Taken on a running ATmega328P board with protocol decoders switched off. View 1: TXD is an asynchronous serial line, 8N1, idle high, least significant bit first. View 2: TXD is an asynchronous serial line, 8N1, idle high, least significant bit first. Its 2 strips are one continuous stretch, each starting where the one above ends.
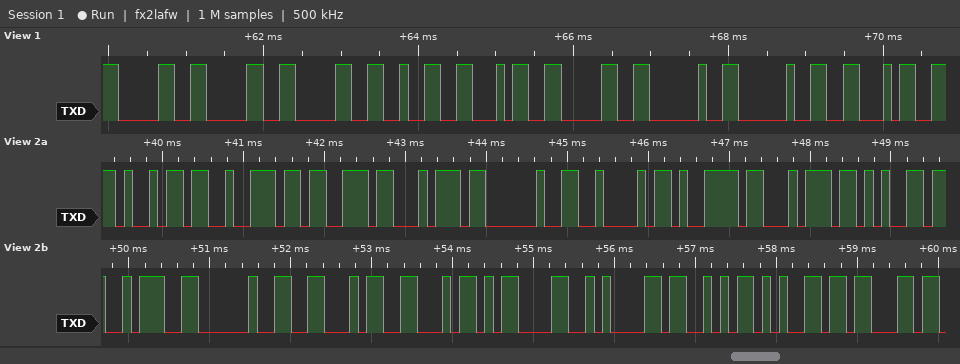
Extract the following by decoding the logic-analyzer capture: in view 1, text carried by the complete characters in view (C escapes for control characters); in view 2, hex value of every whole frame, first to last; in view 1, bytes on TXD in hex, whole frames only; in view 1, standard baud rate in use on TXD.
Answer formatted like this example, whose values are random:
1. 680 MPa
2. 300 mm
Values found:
1. "000240  F"
2. 69 72 73 74 20 42 79 74 65 3A 20 46 46 0D 0A 53 65 63
3. 30 30 30 32 34 30 20 20 46
4. 9600 baud
